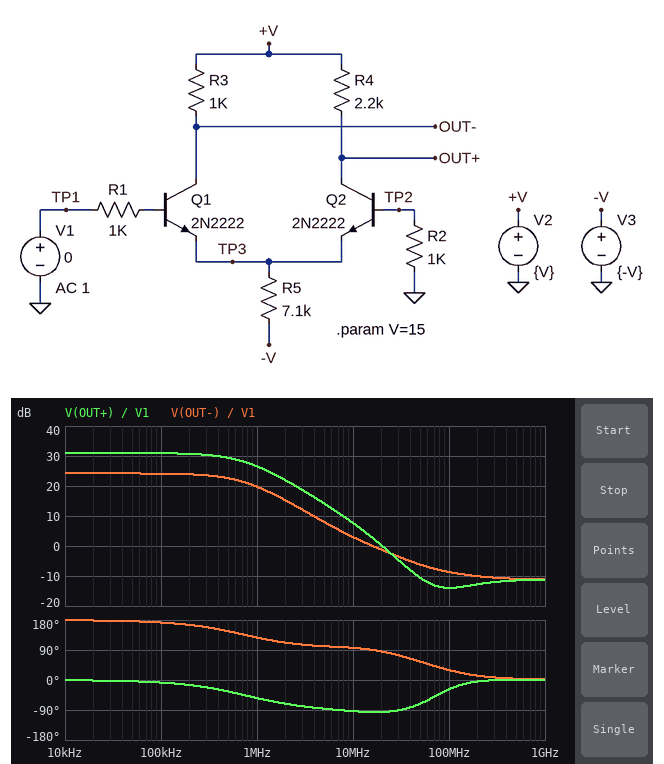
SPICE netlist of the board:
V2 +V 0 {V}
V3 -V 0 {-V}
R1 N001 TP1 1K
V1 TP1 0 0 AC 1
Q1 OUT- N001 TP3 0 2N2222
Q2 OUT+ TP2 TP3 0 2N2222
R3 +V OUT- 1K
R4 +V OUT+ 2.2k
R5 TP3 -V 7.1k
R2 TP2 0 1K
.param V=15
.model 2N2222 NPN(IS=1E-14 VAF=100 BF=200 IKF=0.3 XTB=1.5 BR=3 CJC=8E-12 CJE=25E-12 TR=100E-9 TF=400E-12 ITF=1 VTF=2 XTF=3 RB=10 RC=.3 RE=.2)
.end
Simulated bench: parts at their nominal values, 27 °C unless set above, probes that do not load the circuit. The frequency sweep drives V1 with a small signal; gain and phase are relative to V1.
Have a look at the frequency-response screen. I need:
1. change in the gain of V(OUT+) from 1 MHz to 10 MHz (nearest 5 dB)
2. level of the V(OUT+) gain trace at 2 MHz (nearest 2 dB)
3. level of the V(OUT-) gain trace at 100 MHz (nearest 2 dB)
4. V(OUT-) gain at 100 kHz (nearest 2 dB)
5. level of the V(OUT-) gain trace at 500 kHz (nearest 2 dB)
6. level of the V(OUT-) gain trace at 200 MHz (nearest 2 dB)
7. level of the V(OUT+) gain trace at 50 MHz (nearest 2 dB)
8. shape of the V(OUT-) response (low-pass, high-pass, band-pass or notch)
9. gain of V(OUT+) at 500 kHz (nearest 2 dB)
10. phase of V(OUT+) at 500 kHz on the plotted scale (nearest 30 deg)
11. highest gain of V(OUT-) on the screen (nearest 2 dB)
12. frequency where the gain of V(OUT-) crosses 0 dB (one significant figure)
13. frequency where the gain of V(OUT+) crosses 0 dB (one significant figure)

-20 dB
22 dB
-8 dB
24 dB
22 dB
-10 dB
-10 dB
low-pass
30 dB
-30 deg
24 dB
20 MHz
20 MHz
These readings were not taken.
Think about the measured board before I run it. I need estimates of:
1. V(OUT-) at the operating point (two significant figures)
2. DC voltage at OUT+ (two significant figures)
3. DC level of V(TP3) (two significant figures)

14 V
13 V
-660 mV
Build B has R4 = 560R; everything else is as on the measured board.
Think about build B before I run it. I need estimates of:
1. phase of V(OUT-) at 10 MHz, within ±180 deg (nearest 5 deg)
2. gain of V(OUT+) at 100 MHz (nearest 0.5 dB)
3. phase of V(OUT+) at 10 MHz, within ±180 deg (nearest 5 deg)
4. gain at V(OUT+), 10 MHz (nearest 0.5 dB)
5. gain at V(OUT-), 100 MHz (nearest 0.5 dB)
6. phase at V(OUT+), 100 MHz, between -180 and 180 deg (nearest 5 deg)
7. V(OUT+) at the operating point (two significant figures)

90 deg
-18.5 dB
-85 deg
0.5 dB
-9.0 dB
-20 deg
14 V
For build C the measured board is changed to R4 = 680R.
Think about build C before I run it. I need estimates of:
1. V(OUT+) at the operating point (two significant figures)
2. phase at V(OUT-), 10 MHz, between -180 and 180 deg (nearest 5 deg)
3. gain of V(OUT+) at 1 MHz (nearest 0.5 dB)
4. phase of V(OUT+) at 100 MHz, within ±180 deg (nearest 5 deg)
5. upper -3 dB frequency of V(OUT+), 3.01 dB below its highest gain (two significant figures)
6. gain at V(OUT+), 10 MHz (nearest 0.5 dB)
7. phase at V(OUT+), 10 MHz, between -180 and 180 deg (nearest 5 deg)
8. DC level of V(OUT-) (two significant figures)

14 V
90 deg
18.5 dB
-20 deg
1.2 MHz
2.0 dB
-85 deg
14 V
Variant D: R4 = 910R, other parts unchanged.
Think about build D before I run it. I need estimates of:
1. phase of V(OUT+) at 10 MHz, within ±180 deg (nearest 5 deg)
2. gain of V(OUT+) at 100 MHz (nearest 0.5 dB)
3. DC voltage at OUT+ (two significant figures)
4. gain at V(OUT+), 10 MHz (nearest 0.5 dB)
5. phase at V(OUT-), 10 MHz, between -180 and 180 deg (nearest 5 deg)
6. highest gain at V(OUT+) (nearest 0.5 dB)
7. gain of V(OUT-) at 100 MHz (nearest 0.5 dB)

-85 deg
-16.5 dB
14 V
3.5 dB
90 deg
23.5 dB
-9.0 dB
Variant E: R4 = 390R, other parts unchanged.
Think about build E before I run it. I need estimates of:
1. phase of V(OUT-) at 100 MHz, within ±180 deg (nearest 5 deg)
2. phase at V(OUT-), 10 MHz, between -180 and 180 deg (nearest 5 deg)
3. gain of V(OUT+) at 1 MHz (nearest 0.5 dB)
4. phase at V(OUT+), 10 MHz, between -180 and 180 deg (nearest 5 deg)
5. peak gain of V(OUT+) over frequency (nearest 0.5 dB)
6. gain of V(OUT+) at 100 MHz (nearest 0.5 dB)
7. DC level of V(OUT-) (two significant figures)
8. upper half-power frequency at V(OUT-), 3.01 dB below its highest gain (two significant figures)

35 deg
90 deg
14.0 dB
-80 deg
16.0 dB
-20.0 dB
14 V
1.3 MHz
